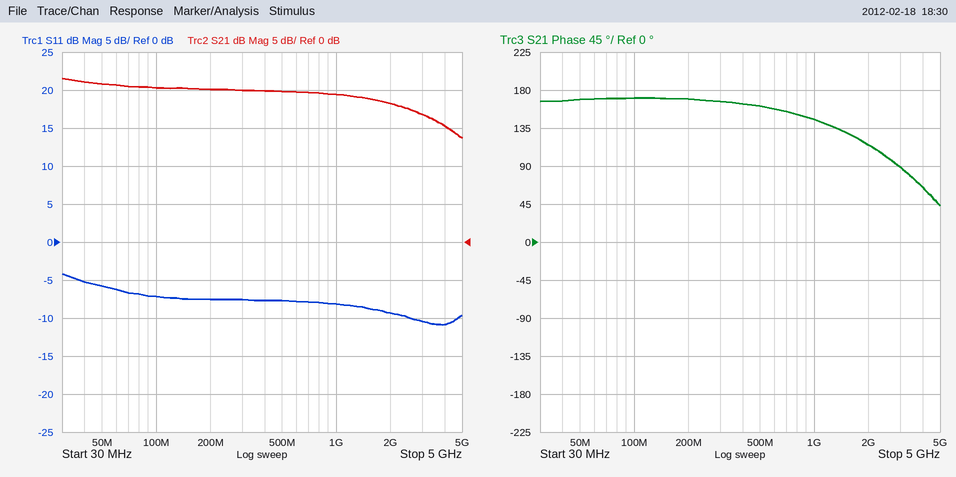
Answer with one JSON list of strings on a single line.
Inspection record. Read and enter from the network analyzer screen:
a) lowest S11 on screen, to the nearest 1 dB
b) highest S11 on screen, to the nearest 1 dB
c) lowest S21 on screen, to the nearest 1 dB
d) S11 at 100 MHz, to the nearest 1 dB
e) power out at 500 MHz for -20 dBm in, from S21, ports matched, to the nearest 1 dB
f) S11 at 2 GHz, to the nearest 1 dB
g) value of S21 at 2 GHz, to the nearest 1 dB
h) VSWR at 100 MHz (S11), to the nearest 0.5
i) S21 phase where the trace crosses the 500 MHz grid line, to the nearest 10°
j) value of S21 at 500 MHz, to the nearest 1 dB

["-11 dB", "-4 dB", "14 dB", "-7 dB", "0 dBm", "-9 dB", "18 dB", "2.5", "160°", "20 dB"]
